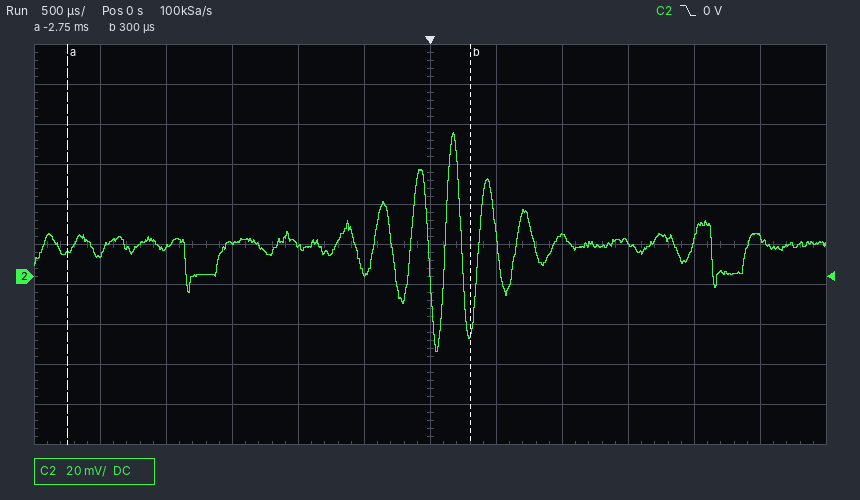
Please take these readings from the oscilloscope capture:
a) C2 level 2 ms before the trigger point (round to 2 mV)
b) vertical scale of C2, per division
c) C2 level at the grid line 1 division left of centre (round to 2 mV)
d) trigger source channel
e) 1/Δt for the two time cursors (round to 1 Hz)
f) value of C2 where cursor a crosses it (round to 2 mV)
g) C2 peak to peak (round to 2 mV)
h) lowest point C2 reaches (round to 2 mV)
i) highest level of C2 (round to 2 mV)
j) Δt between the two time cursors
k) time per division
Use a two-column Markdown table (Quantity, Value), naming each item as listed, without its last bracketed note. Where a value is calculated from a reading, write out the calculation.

| Quantity | Value |
|---|---|
| C2 level 2 ms before the trigger point | 14 mV |
| vertical scale of C2, per division | 20 mV |
| C2 level at the grid line 1 division left of centre | 2 mV |
| trigger source channel | C2 |
| 1/Δt for the two time cursors | 1 / 3.05 ms ≈ 328 Hz |
| value of C2 where cursor a crosses it | 12 mV |
| C2 peak to peak | 72 mV − (-38 mV) = 110 mV |
| lowest point C2 reaches | -38 mV |
| highest level of C2 | 72 mV |
| Δt between the two time cursors | 300 µs − (-2.75 ms) = 3.05 ms |
| time per division | 500 µs |
